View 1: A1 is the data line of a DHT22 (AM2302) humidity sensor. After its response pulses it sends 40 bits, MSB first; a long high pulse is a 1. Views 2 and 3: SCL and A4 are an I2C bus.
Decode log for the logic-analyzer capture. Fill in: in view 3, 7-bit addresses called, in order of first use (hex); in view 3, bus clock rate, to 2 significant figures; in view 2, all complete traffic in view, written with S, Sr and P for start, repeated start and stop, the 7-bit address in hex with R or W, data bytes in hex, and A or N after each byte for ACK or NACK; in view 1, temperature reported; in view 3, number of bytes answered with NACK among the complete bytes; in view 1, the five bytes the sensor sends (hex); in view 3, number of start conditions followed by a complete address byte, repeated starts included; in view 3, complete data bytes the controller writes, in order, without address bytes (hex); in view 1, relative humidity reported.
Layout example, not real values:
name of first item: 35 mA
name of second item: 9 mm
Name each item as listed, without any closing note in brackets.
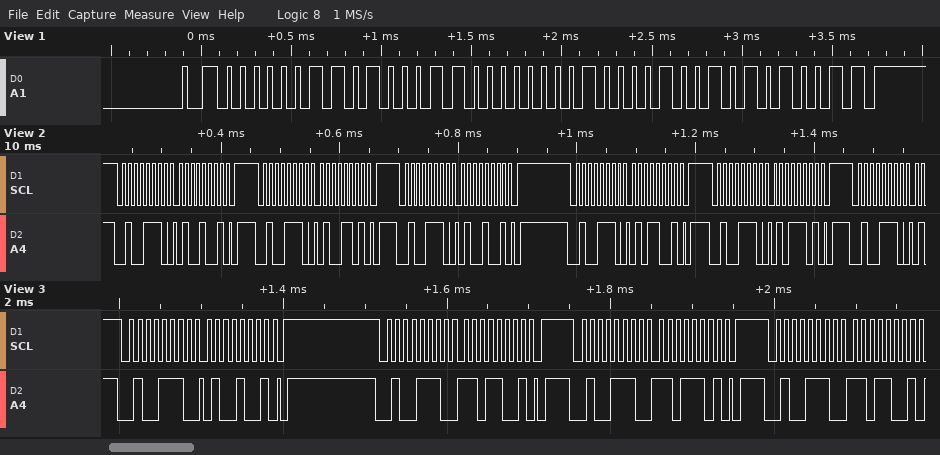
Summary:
in view 3, 7-bit addresses called, in order of first use: 0x27
in view 3, bus clock rate, to 2 significant figures: 100 kHz
in view 2, all complete traffic in view, written with S, Sr and P for start, repeated start and stop, the 7-bit address in hex with R or W, data bytes in hex, and A or N after each byte for ACK or NACK: S 27W A 49 A P S 27W A 4D A P S 27W A 49 A P S 27W A 59 A P S 27W A 5D A P S 27W A
in view 1, temperature reported: 26.5 °C
in view 3, number of bytes answered with NACK among the complete bytes: 0
in view 1, the five bytes the sensor sends: 03 46 01 09 53
in view 3, number of start conditions followed by a complete address byte, repeated starts included: 4
in view 3, complete data bytes the controller writes, in order, without address bytes: 49 D9 DD D9
in view 1, relative humidity reported: 83.8 %
